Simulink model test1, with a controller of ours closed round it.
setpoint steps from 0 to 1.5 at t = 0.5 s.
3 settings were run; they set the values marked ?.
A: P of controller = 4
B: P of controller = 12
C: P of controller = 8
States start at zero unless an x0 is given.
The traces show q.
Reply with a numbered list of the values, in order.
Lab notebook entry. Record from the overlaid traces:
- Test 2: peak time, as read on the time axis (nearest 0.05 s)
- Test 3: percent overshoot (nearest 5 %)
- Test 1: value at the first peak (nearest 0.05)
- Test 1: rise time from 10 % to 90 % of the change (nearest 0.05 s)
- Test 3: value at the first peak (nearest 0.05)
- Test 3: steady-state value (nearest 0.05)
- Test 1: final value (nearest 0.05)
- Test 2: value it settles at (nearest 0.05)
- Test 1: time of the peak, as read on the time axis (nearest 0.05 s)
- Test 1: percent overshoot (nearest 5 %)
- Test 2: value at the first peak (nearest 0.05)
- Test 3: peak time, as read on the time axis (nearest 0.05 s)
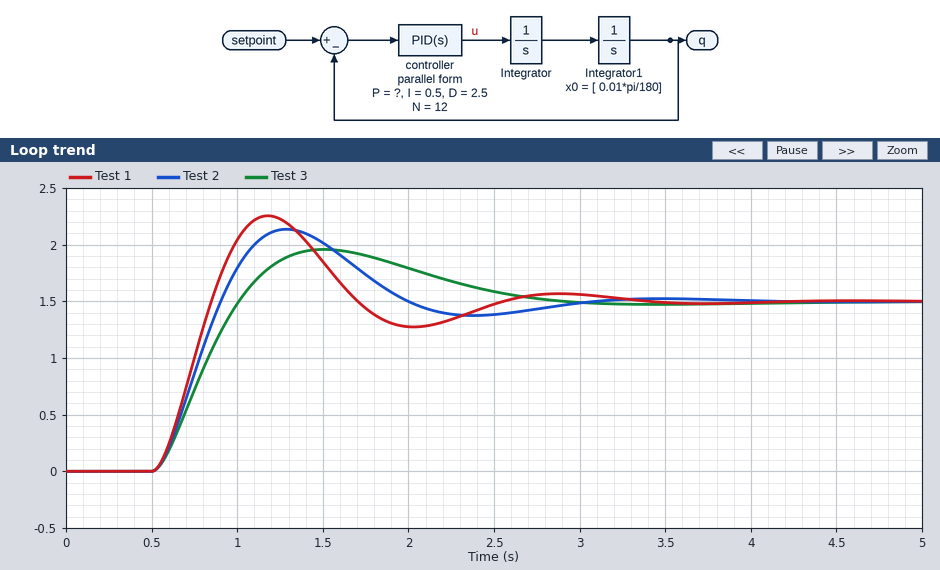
1. 1.30 s
2. 30 %
3. 2.25
4. 0.25 s
5. 1.95
6. 1.50
7. 1.50
8. 1.50
9. 1.20 s
10. 50 %
11. 2.15
12. 1.50 s
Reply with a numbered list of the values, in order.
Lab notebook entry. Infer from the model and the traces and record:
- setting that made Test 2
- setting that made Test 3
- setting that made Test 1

1. C
2. A
3. B
